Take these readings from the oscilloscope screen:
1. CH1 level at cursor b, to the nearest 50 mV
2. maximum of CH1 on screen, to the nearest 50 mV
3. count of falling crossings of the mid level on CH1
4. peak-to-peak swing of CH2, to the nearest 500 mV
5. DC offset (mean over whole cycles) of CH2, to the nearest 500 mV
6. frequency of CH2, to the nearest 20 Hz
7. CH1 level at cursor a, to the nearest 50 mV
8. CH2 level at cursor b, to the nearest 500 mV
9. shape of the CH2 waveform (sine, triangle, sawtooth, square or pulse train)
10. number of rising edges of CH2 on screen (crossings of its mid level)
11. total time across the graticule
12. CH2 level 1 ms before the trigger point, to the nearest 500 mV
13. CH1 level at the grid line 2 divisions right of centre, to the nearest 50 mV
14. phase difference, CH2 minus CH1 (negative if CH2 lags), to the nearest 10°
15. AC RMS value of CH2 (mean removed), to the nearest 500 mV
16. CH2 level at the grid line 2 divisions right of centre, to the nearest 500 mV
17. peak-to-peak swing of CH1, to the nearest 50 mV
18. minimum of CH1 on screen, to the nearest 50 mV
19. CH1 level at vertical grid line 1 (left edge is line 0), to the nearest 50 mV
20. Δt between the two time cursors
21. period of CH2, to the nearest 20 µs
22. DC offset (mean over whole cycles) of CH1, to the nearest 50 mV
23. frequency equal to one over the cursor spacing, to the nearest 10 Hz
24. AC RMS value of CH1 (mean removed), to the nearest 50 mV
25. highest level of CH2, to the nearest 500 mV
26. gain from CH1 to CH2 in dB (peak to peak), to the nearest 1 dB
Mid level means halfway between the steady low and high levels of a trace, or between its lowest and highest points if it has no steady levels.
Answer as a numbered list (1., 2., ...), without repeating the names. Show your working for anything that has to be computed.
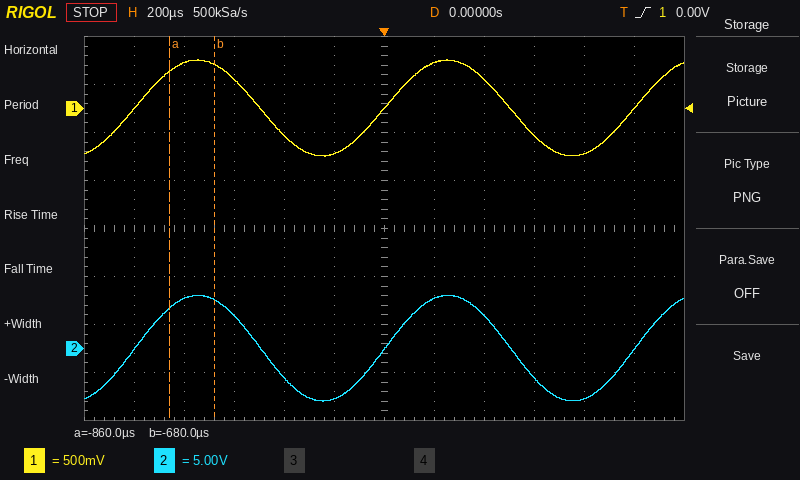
1. 450 mV
2. 500 mV
3. 2
4. 5.5 V − (-5.5 V) = 11.0 V
5. (5.5 V + (-5.5 V)) / 2 ≈ 0.0 V
6. 1 / 1.00 ms ≈ 1.00 kHz
7. 400 mV
8. 5.0 V
9. sine
10. 3
11. 2.4 ms
12. 0.0 V
13. 300 mV
14. −360° × (0 µs) / 1.00 ms ≈ 0°
15. 11.0 V / (2√2) ≈ 3.89 V, so 4.0 V to the nearest 500 mV
16. 3.5 V
17. 500 mV − (-500 mV) = 1.00 V
18. -500 mV
19. 0 mV
20. -680 µs − (-860 µs) = 180 µs
21. 1.00 ms
22. (500 mV + (-500 mV)) / 2 ≈ 0 mV
23. 1 / 180 µs ≈ 5.56 kHz
24. 1.00 V / (2√2) ≈ 354 mV, so 350 mV to the nearest 50 mV
25. 5.5 V
26. 20 log10(11.0 V / 1.00 V) ≈ 21 dB
